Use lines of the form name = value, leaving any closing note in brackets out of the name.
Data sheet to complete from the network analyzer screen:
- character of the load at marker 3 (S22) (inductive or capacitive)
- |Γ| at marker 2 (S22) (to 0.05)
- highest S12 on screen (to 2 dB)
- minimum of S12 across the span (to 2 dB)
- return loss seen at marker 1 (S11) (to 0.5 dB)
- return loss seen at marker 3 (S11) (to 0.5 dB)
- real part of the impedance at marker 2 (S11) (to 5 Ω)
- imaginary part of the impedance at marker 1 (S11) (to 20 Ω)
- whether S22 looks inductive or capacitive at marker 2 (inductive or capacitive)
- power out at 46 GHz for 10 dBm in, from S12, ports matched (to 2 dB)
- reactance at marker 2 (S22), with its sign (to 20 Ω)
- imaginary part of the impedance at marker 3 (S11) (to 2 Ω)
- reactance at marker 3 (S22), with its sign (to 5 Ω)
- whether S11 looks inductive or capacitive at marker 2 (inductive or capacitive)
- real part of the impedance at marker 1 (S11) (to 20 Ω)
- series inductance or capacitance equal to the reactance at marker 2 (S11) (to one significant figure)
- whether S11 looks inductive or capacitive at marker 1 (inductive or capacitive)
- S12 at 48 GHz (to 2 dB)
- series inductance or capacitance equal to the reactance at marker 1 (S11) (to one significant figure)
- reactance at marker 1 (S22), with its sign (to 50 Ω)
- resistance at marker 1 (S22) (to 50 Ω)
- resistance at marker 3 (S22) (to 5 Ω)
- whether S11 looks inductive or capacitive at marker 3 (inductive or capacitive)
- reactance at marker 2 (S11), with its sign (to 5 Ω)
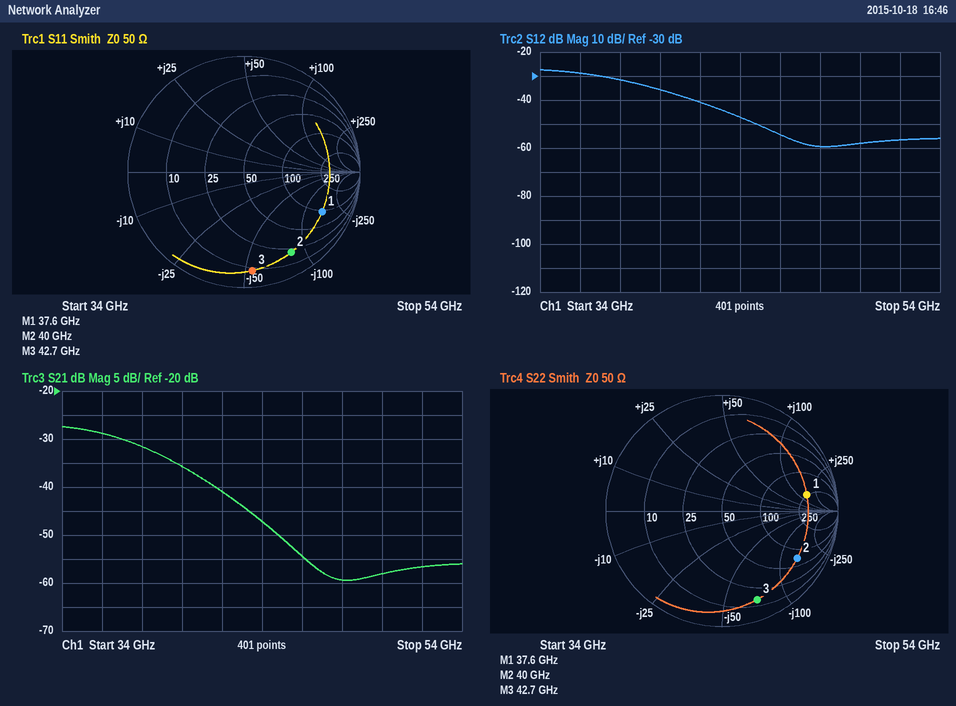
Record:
character of the load at marker 3 (S22) = capacitive
|Γ| at marker 2 (S22) = 0.75
highest S12 on screen = -28 dB
minimum of S12 across the span = -60 dB
return loss seen at marker 1 (S11) = 2.5 dB
return loss seen at marker 3 (S11) = 1.5 dB
real part of the impedance at marker 2 (S11) = 20 Ω
imaginary part of the impedance at marker 1 (S11) = -160 Ω
whether S22 looks inductive or capacitive at marker 2 = capacitive
power out at 46 GHz for 10 dBm in, from S12, ports matched = -44 dBm
reactance at marker 2 (S22), with its sign = -140 Ω
imaginary part of the impedance at marker 3 (S11) = -54 Ω
reactance at marker 3 (S22), with its sign = -70 Ω
whether S11 looks inductive or capacitive at marker 2 = capacitive
real part of the impedance at marker 1 (S11) = 100 Ω
series inductance or capacitance equal to the reactance at marker 2 (S11) = 50 fF
whether S11 looks inductive or capacitive at marker 1 = capacitive
S12 at 48 GHz = -60 dB
series inductance or capacitance equal to the reactance at marker 1 (S11) = 30 fF
reactance at marker 1 (S22), with its sign = +150 Ω
resistance at marker 1 (S22) = 250 Ω
resistance at marker 3 (S22) = 15 Ω
whether S11 looks inductive or capacitive at marker 3 = capacitive
reactance at marker 2 (S11), with its sign = -85 Ω
